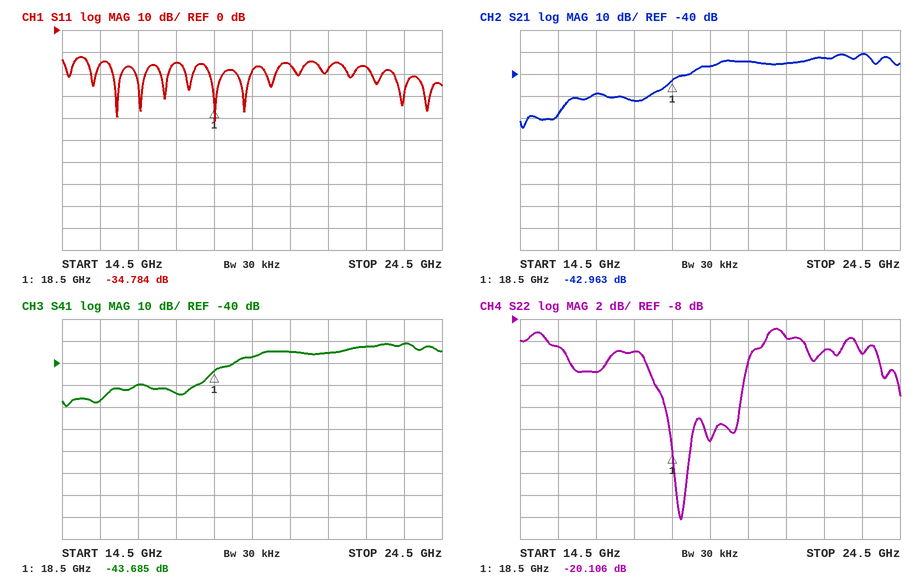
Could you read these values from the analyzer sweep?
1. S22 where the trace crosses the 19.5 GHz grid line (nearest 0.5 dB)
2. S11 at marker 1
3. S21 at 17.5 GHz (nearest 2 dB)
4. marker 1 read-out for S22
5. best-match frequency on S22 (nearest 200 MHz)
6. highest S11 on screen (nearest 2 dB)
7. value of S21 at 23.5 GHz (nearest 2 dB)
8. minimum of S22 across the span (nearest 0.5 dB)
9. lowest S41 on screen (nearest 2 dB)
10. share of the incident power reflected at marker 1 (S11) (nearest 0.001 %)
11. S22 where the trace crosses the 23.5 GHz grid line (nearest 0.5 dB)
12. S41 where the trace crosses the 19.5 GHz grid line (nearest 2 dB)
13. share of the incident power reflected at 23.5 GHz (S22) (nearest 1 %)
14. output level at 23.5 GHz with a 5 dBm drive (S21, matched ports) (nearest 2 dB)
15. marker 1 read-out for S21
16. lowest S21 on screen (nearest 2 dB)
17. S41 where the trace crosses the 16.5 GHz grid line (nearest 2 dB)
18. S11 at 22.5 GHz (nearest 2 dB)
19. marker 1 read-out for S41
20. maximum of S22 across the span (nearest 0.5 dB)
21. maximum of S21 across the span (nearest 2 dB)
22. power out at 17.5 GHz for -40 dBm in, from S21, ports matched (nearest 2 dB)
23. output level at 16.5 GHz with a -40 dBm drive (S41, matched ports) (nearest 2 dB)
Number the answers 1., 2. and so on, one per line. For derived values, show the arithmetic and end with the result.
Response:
1. -19.0 dB
2. -34.784 dB
3. -52 dB
4. -20.106 dB
5. 18.8 GHz
6. -12 dB
7. -30 dB
8. -26.0 dB
9. -60 dB
10. 10^(-34.784/10) ≈ 0.033 %
11. -11.0 dB
12. -38 dB
13. 10^(-11/10) ≈ 8 %
14. 5 dBm + (-30 dB) = -26 dBm
15. -42.963 dB
16. -64 dB
17. -50 dB
18. -16 dB
19. -43.685 dB
20. -9.0 dB
21. -30 dB
22. -40 dBm + (-52 dB) = -92 dBm
23. -40 dBm + (-50 dB) = -90 dBm
